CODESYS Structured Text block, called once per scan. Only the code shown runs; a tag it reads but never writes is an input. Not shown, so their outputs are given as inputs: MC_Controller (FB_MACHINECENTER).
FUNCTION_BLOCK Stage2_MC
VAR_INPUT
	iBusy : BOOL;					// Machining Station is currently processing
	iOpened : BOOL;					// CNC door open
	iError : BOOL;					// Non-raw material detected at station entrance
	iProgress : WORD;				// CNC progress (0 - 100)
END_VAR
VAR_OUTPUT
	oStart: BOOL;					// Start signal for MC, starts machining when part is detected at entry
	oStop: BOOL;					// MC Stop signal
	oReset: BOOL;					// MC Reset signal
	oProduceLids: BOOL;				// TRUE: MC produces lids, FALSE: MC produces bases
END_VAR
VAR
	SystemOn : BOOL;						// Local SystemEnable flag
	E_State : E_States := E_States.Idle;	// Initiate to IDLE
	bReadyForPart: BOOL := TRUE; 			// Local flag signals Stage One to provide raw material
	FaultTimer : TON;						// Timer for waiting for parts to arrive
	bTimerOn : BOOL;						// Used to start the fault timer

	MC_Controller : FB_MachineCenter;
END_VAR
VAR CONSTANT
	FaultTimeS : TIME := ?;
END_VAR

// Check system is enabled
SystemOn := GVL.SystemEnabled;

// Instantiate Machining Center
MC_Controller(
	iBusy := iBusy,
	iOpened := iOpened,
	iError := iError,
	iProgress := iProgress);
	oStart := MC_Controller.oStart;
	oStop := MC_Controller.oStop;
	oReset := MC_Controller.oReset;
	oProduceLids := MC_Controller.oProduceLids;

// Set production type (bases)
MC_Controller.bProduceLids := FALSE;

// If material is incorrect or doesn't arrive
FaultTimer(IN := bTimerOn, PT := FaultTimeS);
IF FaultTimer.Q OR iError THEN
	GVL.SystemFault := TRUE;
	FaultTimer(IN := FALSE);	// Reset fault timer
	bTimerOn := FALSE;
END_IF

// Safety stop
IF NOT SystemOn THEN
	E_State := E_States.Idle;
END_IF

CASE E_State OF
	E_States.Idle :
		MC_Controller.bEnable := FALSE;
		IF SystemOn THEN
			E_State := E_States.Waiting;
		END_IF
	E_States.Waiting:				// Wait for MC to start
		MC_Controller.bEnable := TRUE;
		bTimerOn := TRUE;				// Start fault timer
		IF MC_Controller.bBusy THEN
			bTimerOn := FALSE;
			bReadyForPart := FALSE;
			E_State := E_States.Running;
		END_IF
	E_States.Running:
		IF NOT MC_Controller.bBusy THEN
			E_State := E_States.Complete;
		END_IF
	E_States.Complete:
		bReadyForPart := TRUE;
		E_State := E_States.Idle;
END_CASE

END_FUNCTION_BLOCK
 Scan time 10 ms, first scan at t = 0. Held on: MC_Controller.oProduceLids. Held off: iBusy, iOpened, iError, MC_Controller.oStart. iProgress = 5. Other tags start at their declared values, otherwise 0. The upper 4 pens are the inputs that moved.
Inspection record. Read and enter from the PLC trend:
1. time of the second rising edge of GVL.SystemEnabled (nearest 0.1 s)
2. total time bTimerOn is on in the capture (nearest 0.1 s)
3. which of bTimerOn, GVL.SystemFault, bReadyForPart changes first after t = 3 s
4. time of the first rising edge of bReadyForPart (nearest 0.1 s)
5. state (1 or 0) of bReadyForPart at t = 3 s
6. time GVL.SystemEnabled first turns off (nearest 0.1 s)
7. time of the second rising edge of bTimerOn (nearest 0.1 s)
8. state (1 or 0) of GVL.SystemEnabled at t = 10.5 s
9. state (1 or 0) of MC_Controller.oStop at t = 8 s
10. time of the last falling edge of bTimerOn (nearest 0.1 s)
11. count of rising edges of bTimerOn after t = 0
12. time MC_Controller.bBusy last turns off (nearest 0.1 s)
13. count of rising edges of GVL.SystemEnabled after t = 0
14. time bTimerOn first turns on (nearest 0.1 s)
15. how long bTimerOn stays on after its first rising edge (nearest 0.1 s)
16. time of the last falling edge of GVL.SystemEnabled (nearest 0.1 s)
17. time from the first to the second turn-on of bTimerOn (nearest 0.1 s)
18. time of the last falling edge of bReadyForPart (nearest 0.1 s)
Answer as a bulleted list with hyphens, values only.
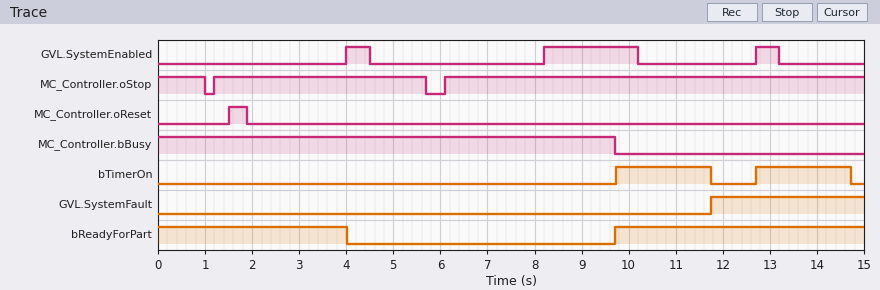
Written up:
- 8.2 s
- 4.0 s
- bReadyForPart
- 9.7 s
- 1
- 4.5 s
- 12.7 s
- 0
- 1
- 14.7 s
- 2
- 9.7 s
- 3
- 9.7 s
- 2.0 s
- 13.2 s
- 3.0 s
- 4.0 s
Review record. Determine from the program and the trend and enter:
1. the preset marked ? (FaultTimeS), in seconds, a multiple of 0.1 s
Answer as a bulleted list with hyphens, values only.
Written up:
- 2.0 s
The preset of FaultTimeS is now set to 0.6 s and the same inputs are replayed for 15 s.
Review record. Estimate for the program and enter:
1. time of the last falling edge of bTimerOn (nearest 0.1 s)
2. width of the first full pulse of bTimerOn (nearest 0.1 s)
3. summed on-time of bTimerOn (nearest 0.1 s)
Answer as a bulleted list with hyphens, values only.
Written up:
- 13.3 s
- 0.6 s
- 1.2 s
